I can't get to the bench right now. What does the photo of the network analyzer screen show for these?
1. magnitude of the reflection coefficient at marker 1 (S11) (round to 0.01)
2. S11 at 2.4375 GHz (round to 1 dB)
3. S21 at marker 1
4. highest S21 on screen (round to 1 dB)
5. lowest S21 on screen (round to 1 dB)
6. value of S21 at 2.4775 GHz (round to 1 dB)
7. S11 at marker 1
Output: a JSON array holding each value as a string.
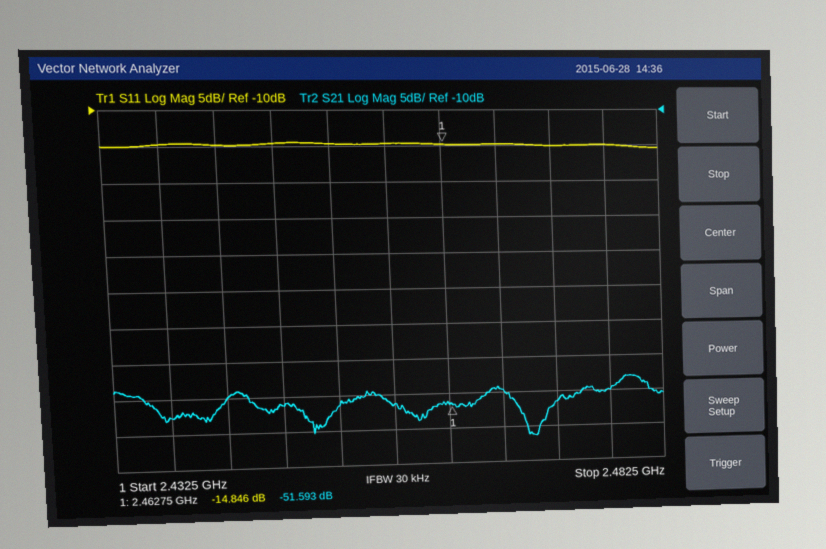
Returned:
["0.18", "-15 dB", "-51.593 dB", "-48 dB", "-56 dB", "-50 dB", "-14.846 dB"]
